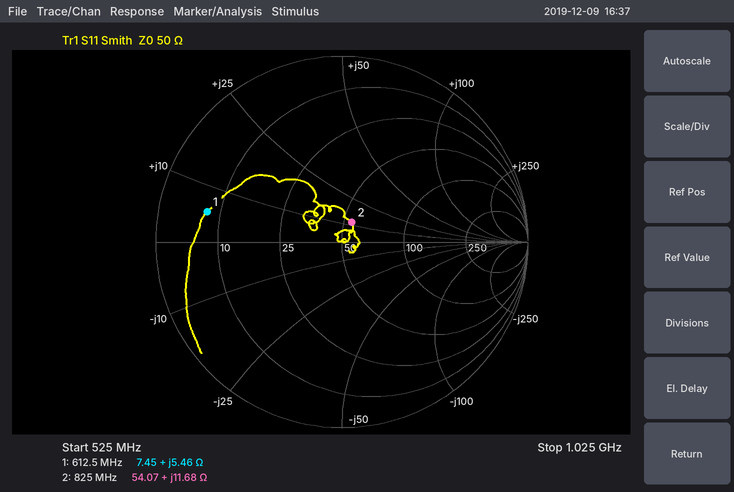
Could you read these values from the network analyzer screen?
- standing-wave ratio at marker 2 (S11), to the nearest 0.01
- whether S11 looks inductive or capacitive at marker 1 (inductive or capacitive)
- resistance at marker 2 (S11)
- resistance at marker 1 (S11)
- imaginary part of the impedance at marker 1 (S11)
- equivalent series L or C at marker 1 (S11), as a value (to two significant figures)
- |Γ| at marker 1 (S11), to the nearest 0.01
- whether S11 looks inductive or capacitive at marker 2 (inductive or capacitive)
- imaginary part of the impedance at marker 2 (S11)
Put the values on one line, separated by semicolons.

1.27; inductive; 54.07 Ω; 7.45 Ω; +5.46 Ω; 1.4 nH; 0.74; inductive; +11.68 Ω
